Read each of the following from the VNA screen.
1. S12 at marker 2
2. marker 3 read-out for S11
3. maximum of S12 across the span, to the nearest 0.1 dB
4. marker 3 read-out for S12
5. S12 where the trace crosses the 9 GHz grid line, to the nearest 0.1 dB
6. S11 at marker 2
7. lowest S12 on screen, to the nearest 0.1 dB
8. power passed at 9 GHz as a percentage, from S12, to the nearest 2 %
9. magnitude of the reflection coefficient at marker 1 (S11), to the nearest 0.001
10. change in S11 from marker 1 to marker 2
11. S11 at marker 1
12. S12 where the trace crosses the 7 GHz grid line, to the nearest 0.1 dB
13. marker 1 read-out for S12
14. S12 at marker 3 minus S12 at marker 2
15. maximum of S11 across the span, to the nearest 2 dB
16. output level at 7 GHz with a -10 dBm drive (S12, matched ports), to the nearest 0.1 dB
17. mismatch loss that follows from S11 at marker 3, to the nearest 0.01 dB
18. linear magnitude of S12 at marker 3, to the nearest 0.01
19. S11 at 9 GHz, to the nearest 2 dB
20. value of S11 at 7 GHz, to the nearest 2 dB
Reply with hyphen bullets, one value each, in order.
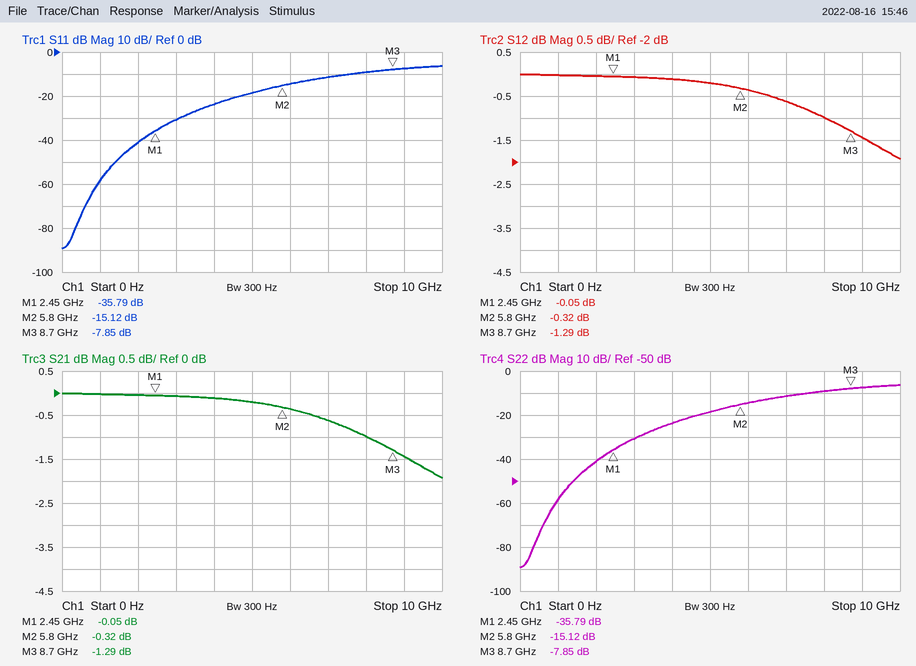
- -0.32 dB
- -7.85 dB
- 0.0 dB
- -1.29 dB
- -1.4 dB
- -15.12 dB
- -1.9 dB
- 72 %
- 0.016
- 20.67 dB
- -35.79 dB
- -0.6 dB
- -0.05 dB
- -0.97 dB
- -6 dB
- -10.6 dBm
- 0.78 dB
- 0.86
- -8 dB
- -12 dB
